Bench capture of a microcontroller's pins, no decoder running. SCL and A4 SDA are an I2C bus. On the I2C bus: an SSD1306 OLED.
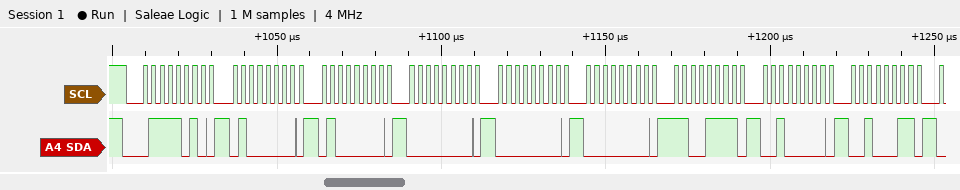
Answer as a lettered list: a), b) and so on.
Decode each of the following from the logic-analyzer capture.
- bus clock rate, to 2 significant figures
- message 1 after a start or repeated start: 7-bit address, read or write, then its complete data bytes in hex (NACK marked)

a) 400 kHz
b) 0x3D write: 40 40 00 00 00 CF 20 23
